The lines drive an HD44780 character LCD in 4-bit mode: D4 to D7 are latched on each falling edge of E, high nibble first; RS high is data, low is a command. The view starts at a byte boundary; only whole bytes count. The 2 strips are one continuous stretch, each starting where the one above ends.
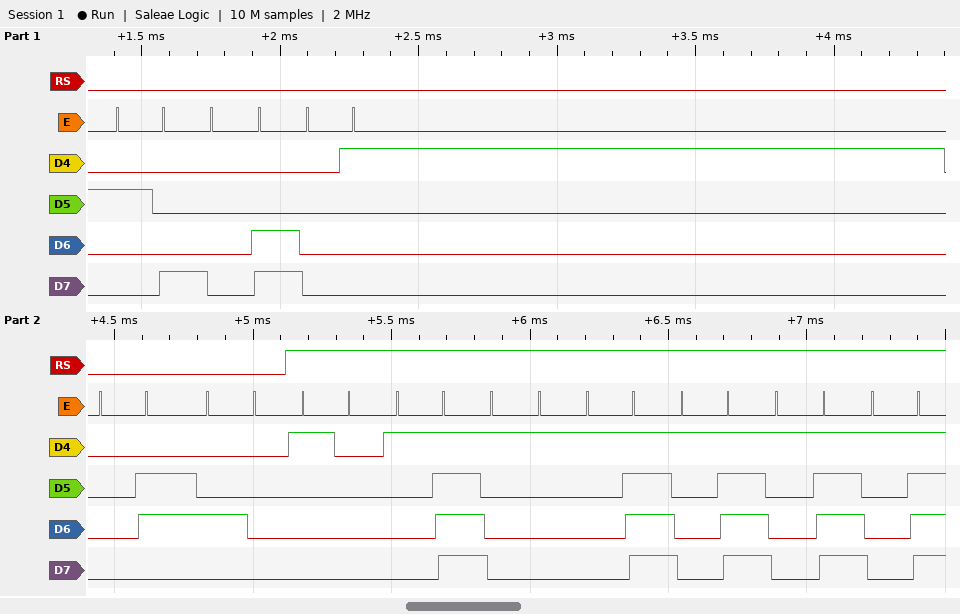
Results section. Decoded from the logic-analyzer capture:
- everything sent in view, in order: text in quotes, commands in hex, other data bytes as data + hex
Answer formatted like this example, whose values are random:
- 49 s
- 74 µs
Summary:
- 0x28 0x0C 0x01 0x06 0x40 data 10 1F 11 1F 1F 1F 1F
